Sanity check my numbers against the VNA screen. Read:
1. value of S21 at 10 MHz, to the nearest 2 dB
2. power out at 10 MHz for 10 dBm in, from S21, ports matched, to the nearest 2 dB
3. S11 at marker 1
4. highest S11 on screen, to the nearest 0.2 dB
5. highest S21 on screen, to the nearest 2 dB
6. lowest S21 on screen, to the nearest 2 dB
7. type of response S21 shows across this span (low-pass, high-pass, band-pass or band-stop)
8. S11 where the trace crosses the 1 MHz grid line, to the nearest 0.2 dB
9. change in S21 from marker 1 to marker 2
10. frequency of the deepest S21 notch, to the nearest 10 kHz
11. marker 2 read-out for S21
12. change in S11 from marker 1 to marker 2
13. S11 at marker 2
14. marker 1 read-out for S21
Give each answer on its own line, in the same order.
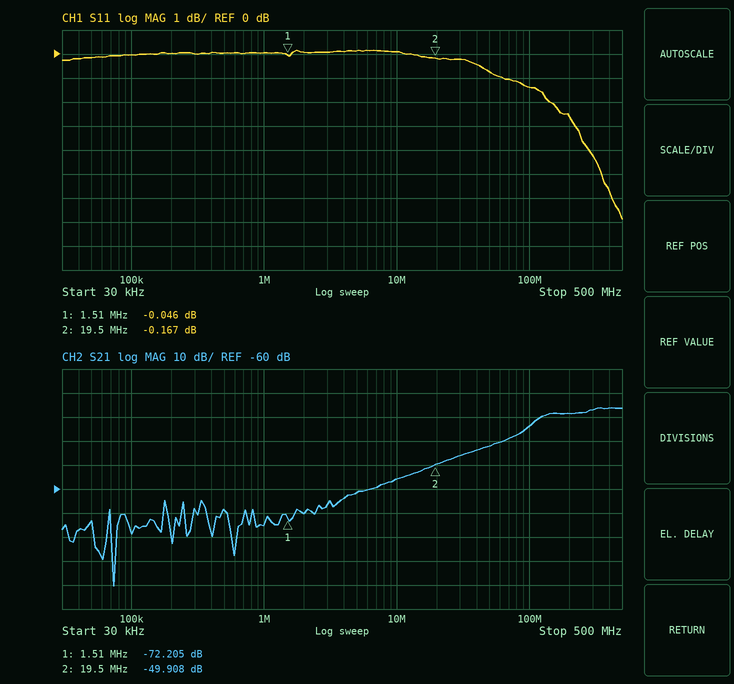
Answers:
-56 dB
-46 dBm
-0.046 dB
0.2 dB
-26 dB
-100 dB
high-pass
0.0 dB
22.297 dB
70 kHz
-49.908 dB
-0.121 dB
-0.167 dB
-72.205 dB
